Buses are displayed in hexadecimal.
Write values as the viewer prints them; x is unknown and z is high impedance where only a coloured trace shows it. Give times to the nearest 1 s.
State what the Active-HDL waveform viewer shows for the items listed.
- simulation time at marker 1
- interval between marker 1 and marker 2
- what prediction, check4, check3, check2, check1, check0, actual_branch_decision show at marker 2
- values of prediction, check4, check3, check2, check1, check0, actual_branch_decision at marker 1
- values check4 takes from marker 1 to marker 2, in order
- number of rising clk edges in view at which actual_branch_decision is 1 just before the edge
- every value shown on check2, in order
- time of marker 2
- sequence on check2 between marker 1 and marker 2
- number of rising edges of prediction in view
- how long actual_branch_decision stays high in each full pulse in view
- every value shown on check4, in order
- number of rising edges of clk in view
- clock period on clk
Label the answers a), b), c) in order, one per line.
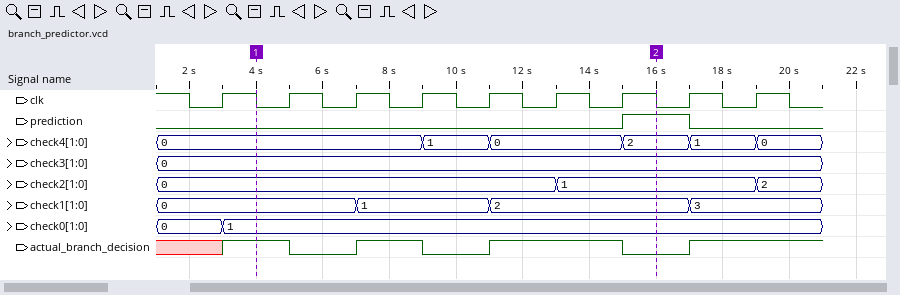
a) 4 s
b) 12 s
c) prediction=1, check4=2, check3=0, check2=1, check1=2, check0=1, actual_branch_decision=0
d) prediction=0, check4=0, check3=0, check2=0, check1=0, check0=1, actual_branch_decision=1
e) 0, 1, 0, 2
f) 5
g) 0, 1, 2
h) 16 s
i) 0, 1
j) 1
k) 2 s, 4 s
l) 0, 1, 0, 2, 1, 0
m) 9
n) 2 s
